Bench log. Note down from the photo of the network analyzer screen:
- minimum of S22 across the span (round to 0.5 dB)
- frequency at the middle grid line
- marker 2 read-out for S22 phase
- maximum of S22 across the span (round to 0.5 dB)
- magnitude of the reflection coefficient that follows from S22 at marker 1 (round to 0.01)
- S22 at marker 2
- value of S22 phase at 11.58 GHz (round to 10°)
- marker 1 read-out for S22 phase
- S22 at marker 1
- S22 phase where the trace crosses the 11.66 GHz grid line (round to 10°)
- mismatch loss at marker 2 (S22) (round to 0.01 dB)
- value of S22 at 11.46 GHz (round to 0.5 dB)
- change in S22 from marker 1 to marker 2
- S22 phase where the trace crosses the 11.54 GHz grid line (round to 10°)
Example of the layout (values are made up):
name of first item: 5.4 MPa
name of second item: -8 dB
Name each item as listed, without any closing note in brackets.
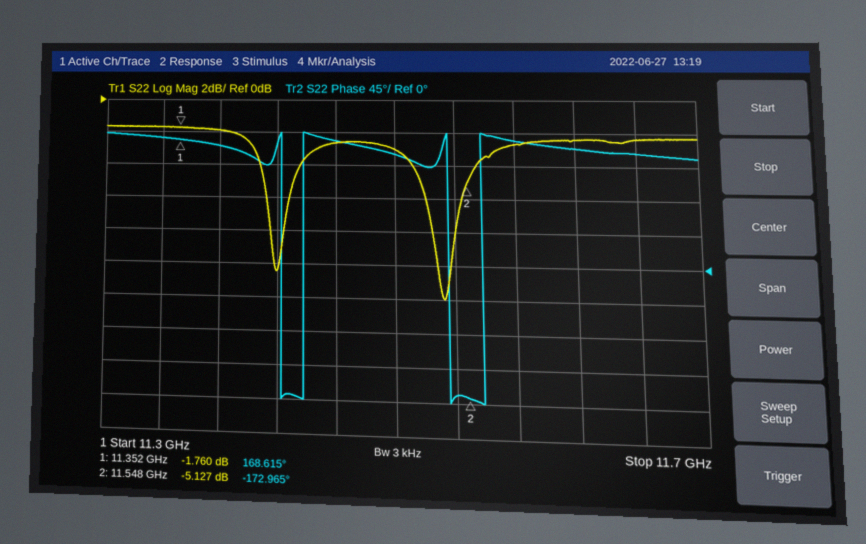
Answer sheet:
minimum of S22 across the span: -12.0 dB
frequency at the middle grid line: 11.5 GHz
marker 2 read-out for S22 phase: -172.965°
maximum of S22 across the span: -1.5 dB
magnitude of the reflection coefficient that follows from S22 at marker 1: 0.82
S22 at marker 2: -5.127 dB
value of S22 phase at 11.58 GHz: 170°
marker 1 read-out for S22 phase: 168.615°
S22 at marker 1: -1.760 dB
S22 phase where the trace crosses the 11.66 GHz grid line: 150°
mismatch loss at marker 2 (S22): 1.59 dB
value of S22 at 11.46 GHz: -2.5 dB
change in S22 from marker 1 to marker 2: -3.367 dB
S22 phase where the trace crosses the 11.54 GHz grid line: -170°
